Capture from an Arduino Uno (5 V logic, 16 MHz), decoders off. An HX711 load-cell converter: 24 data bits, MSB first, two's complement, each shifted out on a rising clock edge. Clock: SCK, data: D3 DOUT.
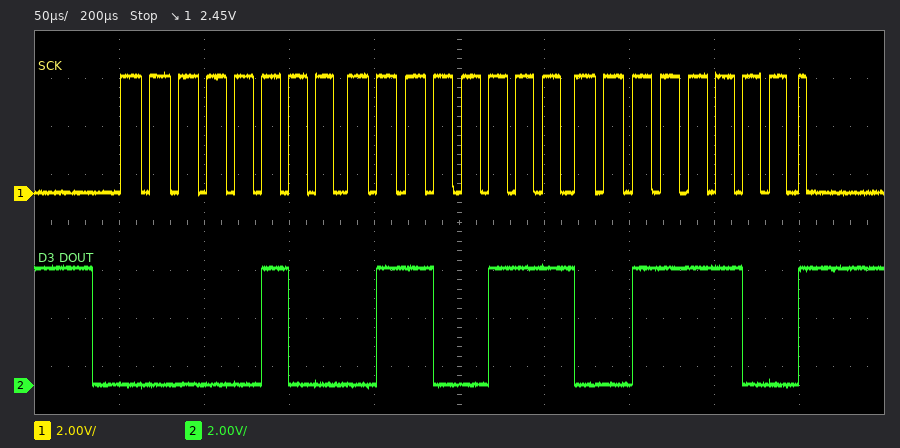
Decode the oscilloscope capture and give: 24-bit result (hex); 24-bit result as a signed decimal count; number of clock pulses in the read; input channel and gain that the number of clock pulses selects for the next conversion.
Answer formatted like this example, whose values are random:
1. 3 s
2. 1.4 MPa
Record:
1. 0x04673C
2. 288572
3. 25
4. channel A, gain 128
